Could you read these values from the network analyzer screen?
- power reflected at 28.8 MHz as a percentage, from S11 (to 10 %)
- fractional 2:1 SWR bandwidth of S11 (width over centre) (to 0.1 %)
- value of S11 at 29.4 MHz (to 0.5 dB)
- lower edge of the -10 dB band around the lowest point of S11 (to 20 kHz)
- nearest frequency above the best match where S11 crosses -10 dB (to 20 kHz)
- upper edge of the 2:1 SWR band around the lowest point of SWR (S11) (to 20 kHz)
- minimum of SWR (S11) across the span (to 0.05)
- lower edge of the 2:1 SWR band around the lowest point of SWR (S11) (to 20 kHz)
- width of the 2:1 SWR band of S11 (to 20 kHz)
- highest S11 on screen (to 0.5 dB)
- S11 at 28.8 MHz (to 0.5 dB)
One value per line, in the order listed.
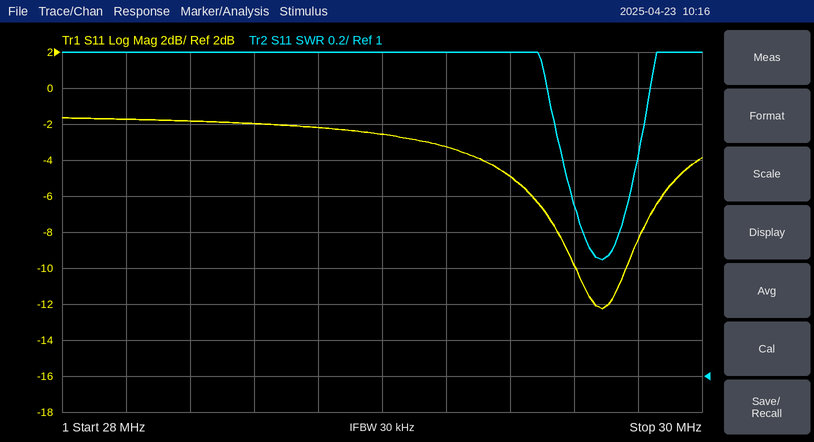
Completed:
60 %
0.6 %
-5.0 dB
29.60 MHz
29.76 MHz
29.78 MHz
1.65
29.60 MHz
180 kHz
-1.5 dB
-2.0 dB
